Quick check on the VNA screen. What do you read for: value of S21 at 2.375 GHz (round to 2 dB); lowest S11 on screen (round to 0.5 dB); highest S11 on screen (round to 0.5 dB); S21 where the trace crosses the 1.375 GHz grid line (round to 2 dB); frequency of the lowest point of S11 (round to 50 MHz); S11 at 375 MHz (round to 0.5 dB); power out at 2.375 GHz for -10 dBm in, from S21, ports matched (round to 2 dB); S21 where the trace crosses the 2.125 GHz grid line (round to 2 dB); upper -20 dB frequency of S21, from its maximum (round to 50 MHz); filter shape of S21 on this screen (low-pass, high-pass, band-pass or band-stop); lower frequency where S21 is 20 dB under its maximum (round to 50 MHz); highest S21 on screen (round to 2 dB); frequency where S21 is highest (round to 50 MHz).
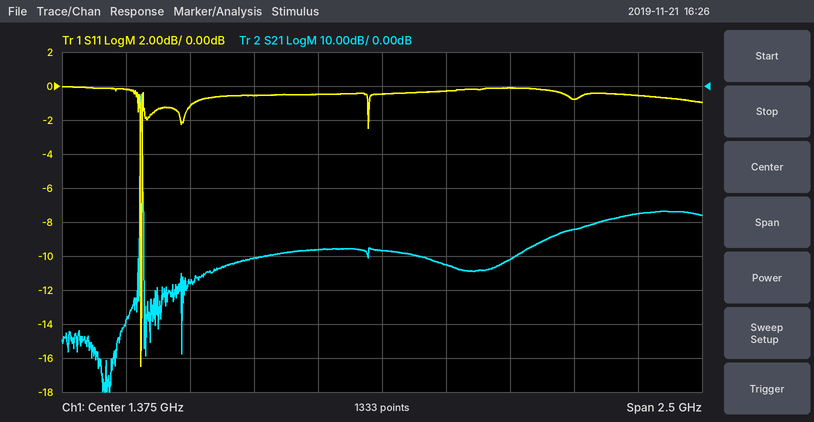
-38 dB
-16.5 dB
0.0 dB
-48 dB
450 MHz
0.0 dB
-48 dBm
-42 dB
450 MHz
band-pass
450 MHz
-2 dB
450 MHz
